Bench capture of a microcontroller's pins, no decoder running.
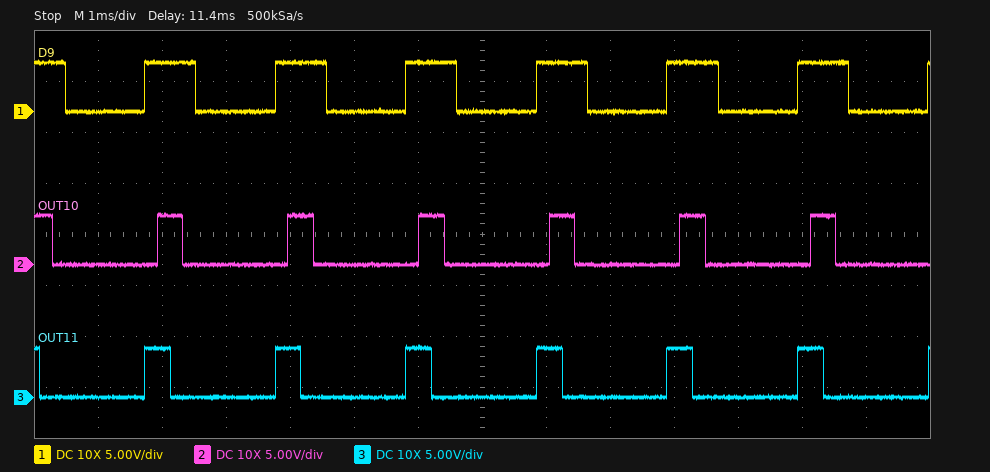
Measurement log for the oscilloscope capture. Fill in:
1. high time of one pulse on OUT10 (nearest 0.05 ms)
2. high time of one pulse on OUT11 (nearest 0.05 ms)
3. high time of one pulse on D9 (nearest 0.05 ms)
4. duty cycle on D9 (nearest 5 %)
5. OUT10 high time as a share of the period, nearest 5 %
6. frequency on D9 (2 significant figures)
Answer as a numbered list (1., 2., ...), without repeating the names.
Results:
1. 0.40 ms
2. 0.40 ms
3. 0.80 ms
4. 40 %
5. 20 %
6. 490 Hz
